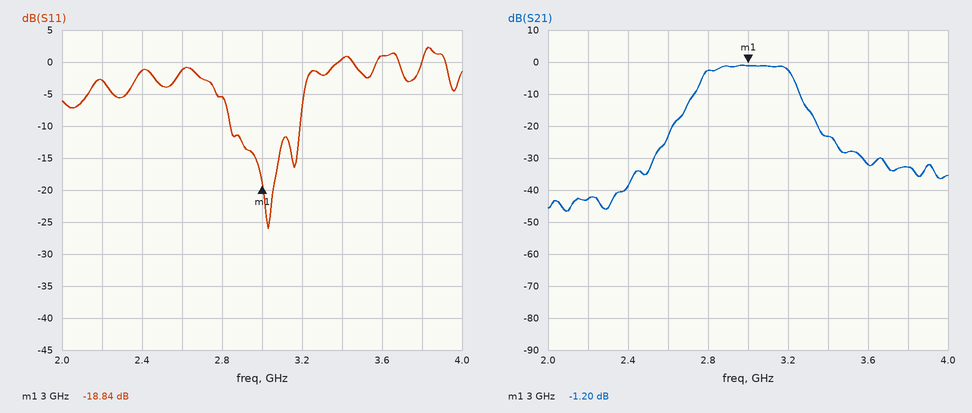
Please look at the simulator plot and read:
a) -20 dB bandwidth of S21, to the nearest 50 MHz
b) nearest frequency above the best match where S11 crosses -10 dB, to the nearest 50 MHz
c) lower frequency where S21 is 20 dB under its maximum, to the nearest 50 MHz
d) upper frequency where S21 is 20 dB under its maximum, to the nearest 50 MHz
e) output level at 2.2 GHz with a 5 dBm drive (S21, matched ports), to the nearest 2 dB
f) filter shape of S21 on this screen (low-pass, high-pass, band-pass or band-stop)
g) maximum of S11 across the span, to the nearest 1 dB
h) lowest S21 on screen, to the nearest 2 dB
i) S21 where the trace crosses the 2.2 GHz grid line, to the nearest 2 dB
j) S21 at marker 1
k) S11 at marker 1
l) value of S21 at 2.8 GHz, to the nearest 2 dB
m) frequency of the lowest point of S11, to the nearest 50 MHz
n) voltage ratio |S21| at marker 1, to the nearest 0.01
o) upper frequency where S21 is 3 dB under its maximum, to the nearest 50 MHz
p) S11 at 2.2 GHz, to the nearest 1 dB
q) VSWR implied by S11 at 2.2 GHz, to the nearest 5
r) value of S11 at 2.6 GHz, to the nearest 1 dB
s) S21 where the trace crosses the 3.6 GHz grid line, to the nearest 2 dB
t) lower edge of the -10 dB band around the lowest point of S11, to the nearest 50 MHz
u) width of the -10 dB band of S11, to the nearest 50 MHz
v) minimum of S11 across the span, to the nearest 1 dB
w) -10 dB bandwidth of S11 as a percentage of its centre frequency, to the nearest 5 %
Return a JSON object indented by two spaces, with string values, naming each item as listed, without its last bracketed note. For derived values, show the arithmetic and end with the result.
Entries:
{
  "-20 dB bandwidth of S21, to the nearest 50 MHz": "3.35 GHz − 2.60 GHz = 750 MHz",
  "nearest frequency above the best match where S11 crosses -10 dB, to the nearest 50 MHz": "3.20 GHz",
  "lower frequency where S21 is 20 dB under its maximum, to the nearest 50 MHz": "2.60 GHz",
  "upper frequency where S21 is 20 dB under its maximum, to the nearest 50 MHz": "3.35 GHz",
  "output level at 2.2 GHz with a 5 dBm drive (S21, matched ports), to the nearest 2 dB": "5 dBm + (-42 dB) = -38 dBm",
  "filter shape of S21 on this screen": "band-pass",
  "maximum of S11 across the span, to the nearest 1 dB": "2 dB",
  "lowest S21 on screen, to the nearest 2 dB": "-46 dB",
  "S21 where the trace crosses the 2.2 GHz grid line, to the nearest 2 dB": "-42 dB",
  "S21 at marker 1": "-1.20 dB",
  "S11 at marker 1": "-18.84 dB",
  "value of S21 at 2.8 GHz, to the nearest 2 dB": "-2 dB",
  "frequency of the lowest point of S11, to the nearest 50 MHz": "3.05 GHz",
  "voltage ratio |S21| at marker 1, to the nearest 0.01": "10^(-1.2/20) ≈ 0.87",
  "upper frequency where S21 is 3 dB under its maximum, to the nearest 50 MHz": "3.20 GHz",
  "S11 at 2.2 GHz, to the nearest 1 dB": "-3 dB",
  "VSWR implied by S11 at 2.2 GHz, to the nearest 5": "|Γ| = 10^(-3/20) = 0.7079; VSWR = (1 + 0.7079)/(1 − 0.7079) ≈ 5.85, so 5 to the nearest 5",
  "value of S11 at 2.6 GHz, to the nearest 1 dB": "-1 dB",
  "S21 where the trace crosses the 3.6 GHz grid line, to the nearest 2 dB": "-32 dB",
  "lower edge of the -10 dB band around the lowest point of S11, to the nearest 50 MHz": "2.85 GHz",
  "width of the -10 dB band of S11, to the nearest 50 MHz": "3.20 GHz − 2.85 GHz = 350 MHz",
  "minimum of S11 across the span, to the nearest 1 dB": "-26 dB",
  "-10 dB bandwidth of S11 as a percentage of its centre frequency, to the nearest 5 %": "350 MHz / 3.025 GHz ≈ 11.6 %, so 10 % to the nearest 5 %"
}
